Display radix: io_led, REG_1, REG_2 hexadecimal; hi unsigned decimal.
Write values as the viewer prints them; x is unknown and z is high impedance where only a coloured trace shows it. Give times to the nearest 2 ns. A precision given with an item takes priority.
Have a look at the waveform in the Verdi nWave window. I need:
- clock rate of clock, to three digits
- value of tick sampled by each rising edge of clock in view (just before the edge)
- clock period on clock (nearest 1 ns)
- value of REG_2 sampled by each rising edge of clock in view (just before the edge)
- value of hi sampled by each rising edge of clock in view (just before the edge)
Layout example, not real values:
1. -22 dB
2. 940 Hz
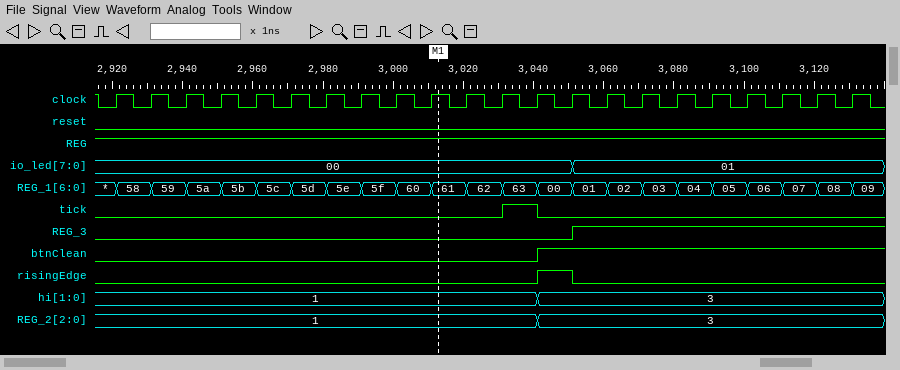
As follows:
1. 100 MHz
2. 0 0 0 0 0 0 0 0 0 0 0 0 1 0 0 0 0 0 0 0 0 0
3. 10 ns
4. 1, 1, 1, 1, 1, 1, 1, 1, 1, 1, 1, 1, 1, 3, 3, 3, 3, 3, 3, 3, 3, 3
5. 1, 1, 1, 1, 1, 1, 1, 1, 1, 1, 1, 1, 1, 3, 3, 3, 3, 3, 3, 3, 3, 3
